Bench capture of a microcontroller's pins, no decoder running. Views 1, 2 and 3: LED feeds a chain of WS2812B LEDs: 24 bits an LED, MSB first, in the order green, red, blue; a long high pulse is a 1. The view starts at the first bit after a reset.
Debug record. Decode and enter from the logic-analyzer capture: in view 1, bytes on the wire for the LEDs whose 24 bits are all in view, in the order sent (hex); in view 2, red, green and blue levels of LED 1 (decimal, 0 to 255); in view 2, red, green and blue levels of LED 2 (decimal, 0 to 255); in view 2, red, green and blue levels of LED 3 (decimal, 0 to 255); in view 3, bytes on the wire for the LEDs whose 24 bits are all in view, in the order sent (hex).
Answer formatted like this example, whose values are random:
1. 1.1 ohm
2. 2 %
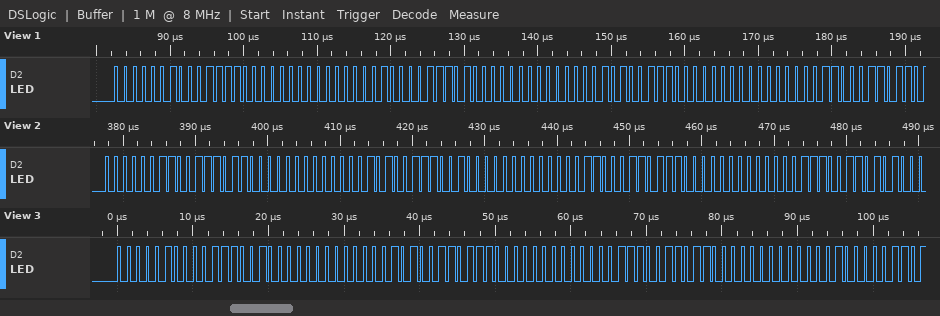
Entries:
1. 02 3C 00 04 3A 00 05 38 00
2. 59, 3, 0
3. 57, 5, 0
4. 55, 6, 0
5. 04 39 00 05 37 00 07 36 00
